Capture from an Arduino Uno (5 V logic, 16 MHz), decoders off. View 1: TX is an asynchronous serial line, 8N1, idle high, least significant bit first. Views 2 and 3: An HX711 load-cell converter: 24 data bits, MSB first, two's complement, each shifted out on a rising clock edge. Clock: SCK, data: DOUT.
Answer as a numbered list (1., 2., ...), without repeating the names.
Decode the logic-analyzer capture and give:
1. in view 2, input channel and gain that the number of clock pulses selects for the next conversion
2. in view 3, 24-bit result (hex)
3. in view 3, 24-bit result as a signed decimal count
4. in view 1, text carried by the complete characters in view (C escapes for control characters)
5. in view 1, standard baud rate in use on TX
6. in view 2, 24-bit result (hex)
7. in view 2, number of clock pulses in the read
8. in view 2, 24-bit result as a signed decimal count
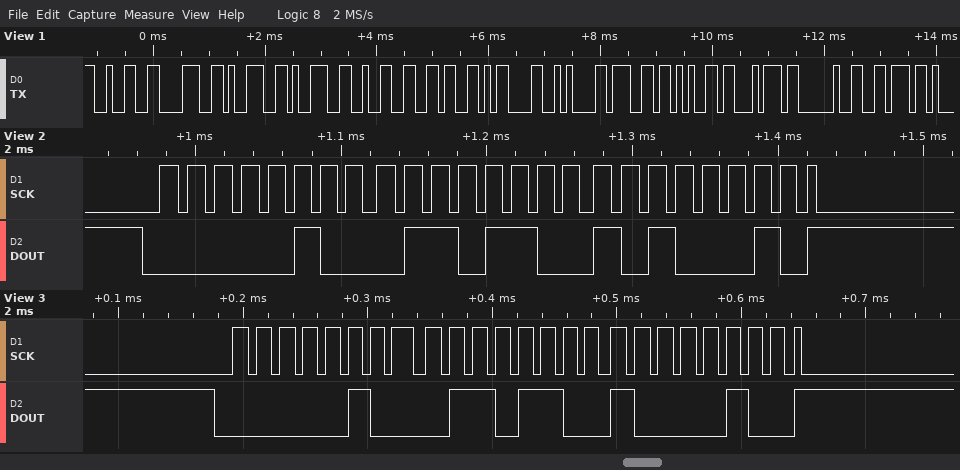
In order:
1. channel A, gain 128
2. 0x046C84
3. 289924
4. "289926\r\nget v"
5. 9600 baud
6. 0x046CA2
7. 25
8. 289954
